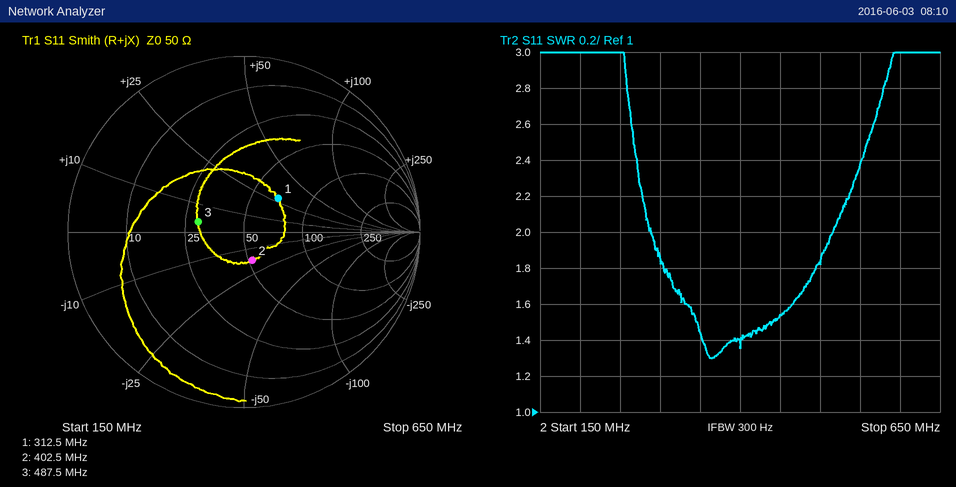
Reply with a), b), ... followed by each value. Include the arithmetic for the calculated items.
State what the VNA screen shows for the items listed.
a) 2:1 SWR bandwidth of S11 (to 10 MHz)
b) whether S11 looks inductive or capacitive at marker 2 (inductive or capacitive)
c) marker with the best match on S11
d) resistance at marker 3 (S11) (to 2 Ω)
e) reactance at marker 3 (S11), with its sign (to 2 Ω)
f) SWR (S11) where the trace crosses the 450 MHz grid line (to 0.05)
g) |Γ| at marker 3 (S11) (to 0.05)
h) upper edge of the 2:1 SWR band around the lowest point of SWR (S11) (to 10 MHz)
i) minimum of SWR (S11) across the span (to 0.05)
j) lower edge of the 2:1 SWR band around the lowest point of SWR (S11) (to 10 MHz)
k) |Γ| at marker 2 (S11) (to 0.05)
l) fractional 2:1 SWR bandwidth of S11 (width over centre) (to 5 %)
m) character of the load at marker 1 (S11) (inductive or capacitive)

a) 520 MHz − 290 MHz = 230 MHz
b) capacitive
c) marker 2
d) 30 Ω
e) +4 Ω
f) 1.55
g) 0.25
h) 520 MHz
i) 1.30
j) 290 MHz
k) 0.15
l) 230 MHz / 405 MHz ≈ 56.8 %, so 55 % to the nearest 5 %
m) inductive
